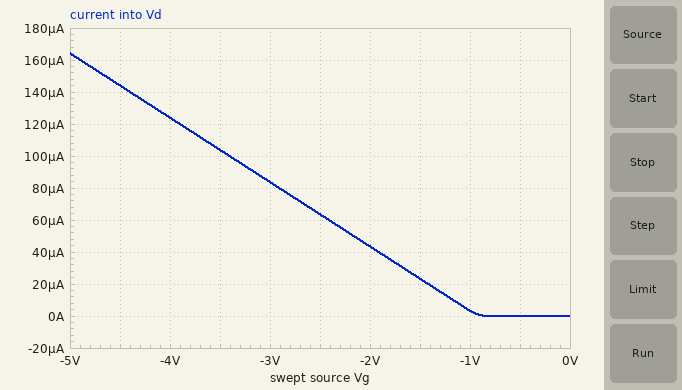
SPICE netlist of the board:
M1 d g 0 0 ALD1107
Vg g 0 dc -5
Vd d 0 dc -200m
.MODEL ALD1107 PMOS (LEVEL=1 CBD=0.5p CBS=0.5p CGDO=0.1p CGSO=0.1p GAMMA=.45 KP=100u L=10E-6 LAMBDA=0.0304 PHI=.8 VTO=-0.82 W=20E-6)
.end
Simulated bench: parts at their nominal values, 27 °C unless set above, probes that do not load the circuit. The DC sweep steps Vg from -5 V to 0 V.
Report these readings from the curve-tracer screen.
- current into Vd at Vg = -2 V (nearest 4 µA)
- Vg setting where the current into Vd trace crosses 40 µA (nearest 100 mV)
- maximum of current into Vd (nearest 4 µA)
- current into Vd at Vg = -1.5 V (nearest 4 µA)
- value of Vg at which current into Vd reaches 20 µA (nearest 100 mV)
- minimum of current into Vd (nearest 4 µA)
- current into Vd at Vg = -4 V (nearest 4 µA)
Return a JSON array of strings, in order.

["44 µA", "-1.9 V", "164 µA", "24 µA", "-1.4 V", "0 A", "124 µA"]
